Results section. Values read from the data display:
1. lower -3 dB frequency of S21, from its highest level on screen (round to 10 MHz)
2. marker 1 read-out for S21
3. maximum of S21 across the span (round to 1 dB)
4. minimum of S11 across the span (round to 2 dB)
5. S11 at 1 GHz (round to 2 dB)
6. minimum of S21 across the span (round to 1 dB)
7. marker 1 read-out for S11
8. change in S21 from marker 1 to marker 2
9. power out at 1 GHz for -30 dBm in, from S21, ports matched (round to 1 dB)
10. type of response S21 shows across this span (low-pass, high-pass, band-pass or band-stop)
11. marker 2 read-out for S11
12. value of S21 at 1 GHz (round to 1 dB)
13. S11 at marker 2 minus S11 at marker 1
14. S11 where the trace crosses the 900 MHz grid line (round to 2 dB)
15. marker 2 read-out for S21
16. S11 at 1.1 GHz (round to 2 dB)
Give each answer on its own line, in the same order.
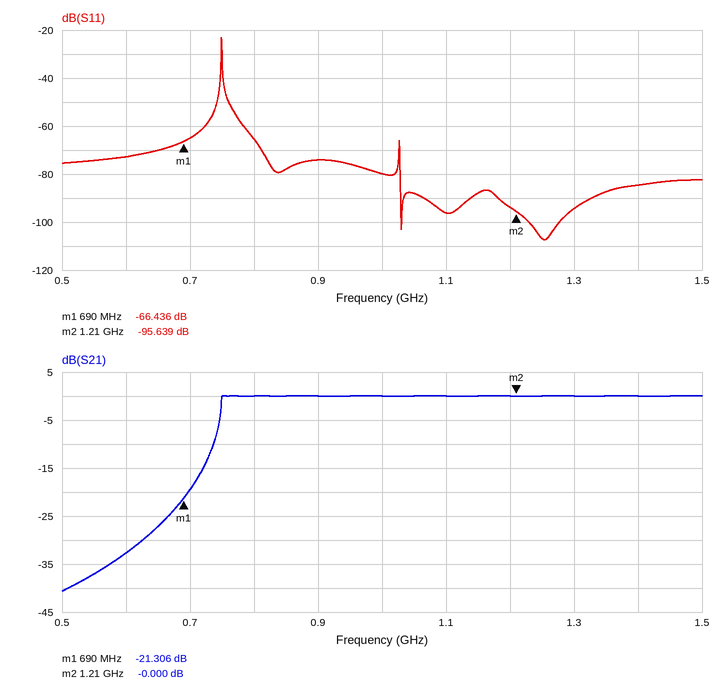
750 MHz
-21.306 dB
0 dB
-108 dB
-80 dB
-41 dB
-66.436 dB
21.306 dB
-30 dBm
high-pass
-95.639 dB
0 dB
-29.203 dB
-74 dB
-0.000 dB
-96 dB
